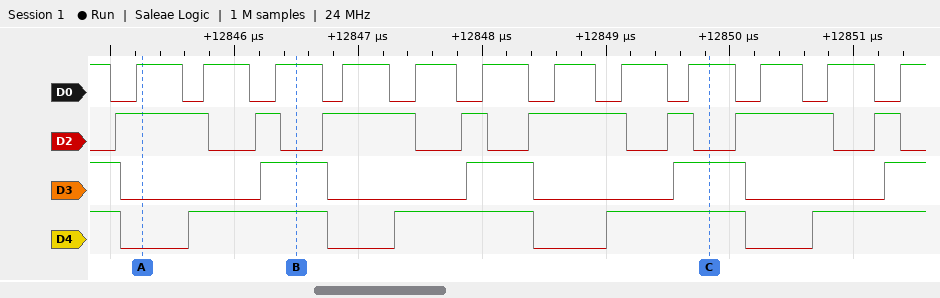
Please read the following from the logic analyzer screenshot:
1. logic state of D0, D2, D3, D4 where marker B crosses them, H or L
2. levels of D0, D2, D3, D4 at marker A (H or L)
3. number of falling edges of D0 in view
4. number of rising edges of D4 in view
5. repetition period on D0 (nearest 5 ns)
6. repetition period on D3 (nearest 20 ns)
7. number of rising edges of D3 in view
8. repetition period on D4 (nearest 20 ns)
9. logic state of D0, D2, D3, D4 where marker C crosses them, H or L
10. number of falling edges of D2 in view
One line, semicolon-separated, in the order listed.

D0=H, D2=L, D3=H, D4=H; D0=H, D2=H, D3=L, D4=L; 12; 4; 560 ns; 1680 ns; 4; 1680 ns; D0=H, D2=L, D3=H, D4=H; 8
